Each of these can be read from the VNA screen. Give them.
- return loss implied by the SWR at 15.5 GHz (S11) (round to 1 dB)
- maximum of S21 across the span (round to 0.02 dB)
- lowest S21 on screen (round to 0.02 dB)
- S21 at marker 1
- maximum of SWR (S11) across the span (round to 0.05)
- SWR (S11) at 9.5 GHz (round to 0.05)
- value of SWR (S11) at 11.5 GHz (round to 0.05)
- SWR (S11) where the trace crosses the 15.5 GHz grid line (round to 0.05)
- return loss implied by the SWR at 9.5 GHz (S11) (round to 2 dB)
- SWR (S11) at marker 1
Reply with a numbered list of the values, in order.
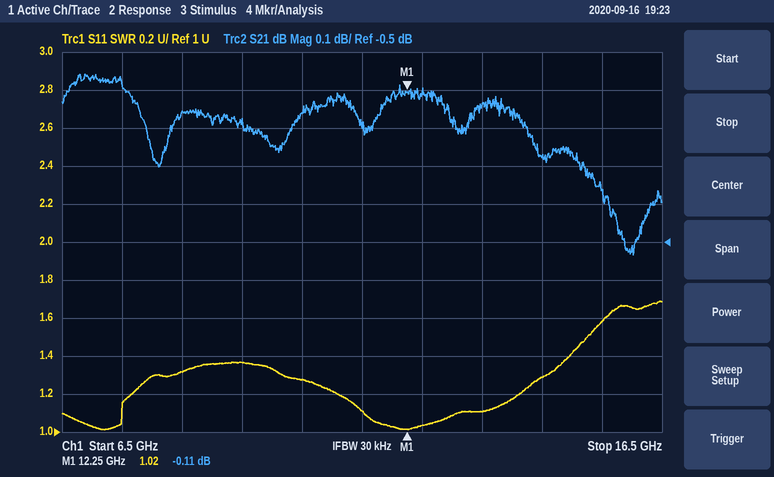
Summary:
1. 13 dB
2. -0.06 dB
3. -0.54 dB
4. -0.11 dB
5. 1.70
6. 1.35
7. 1.10
8. 1.60
9. 16 dB
10. 1.02
